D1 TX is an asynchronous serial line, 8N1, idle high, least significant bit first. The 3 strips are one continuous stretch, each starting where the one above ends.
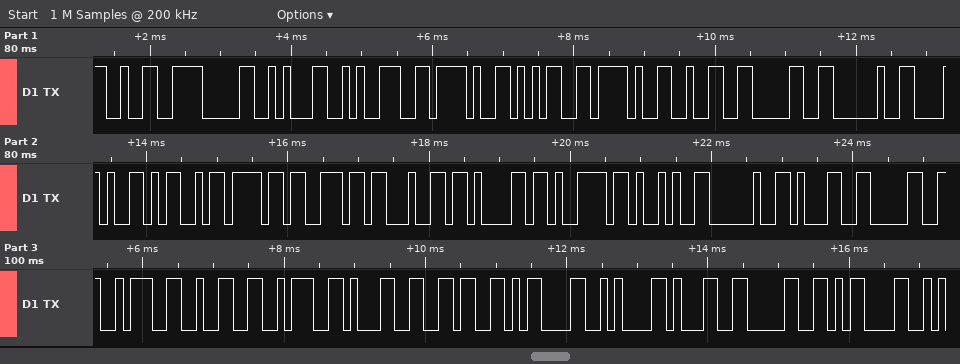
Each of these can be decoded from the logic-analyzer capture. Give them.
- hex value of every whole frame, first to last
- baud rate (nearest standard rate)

32 30 31 39 2F 35 2F 32 30 20 28 4D 6F 6E 64 61 79 29 20 31 30 3A 32 3A 31 36 0D 0A 31 30 0D
9600 baud
